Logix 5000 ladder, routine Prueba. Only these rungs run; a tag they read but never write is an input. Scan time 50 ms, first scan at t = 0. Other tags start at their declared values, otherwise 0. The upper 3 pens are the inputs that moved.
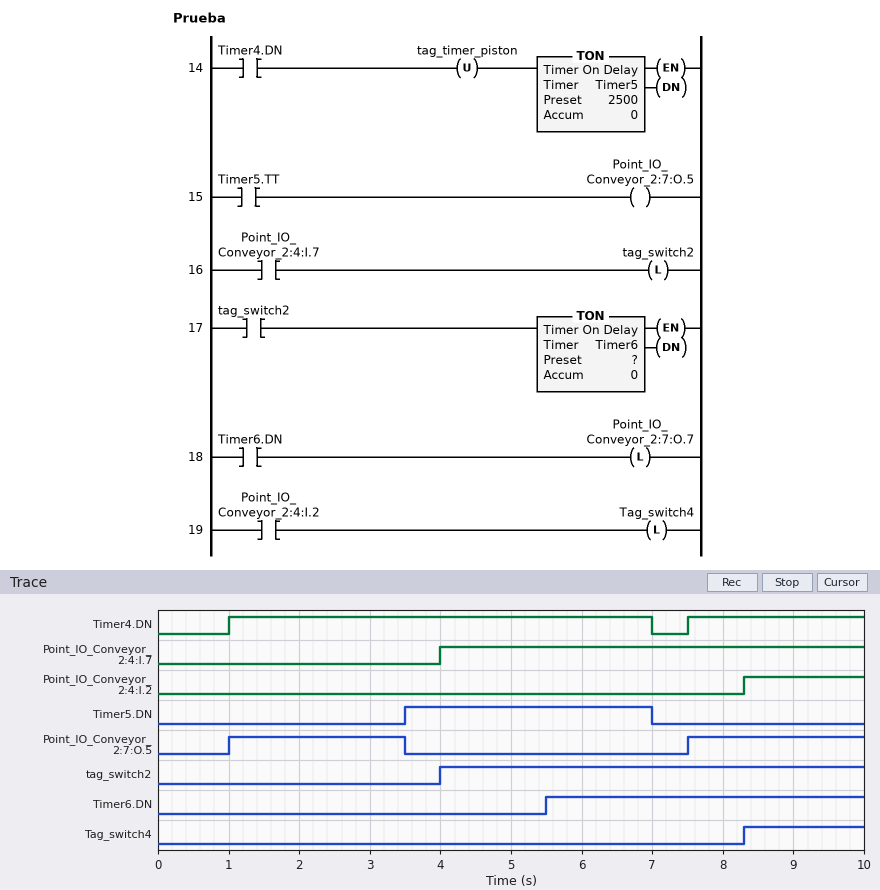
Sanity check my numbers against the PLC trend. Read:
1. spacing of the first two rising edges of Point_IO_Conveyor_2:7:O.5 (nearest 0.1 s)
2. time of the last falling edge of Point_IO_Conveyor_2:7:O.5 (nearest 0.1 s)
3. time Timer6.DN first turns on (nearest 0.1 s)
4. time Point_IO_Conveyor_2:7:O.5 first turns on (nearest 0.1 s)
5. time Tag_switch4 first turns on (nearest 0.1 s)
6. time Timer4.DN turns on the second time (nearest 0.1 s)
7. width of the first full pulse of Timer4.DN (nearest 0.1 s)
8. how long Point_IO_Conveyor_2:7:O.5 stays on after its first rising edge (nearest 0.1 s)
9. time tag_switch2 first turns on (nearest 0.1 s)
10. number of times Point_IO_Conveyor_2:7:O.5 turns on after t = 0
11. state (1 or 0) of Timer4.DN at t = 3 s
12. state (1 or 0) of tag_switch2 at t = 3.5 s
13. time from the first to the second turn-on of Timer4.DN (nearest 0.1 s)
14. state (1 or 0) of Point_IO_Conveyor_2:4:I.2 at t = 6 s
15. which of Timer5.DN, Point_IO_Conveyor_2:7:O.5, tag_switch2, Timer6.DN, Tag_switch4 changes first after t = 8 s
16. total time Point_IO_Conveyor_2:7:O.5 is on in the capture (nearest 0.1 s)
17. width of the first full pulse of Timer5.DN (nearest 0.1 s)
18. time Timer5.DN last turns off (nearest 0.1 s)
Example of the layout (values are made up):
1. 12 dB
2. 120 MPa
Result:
1. 6.5 s
2. 3.5 s
3. 5.5 s
4. 1.0 s
5. 8.3 s
6. 7.5 s
7. 6.0 s
8. 2.5 s
9. 4.0 s
10. 2
11. 1
12. 0
13. 6.5 s
14. 0
15. Tag_switch4
16. 5.0 s
17. 3.5 s
18. 7.0 s
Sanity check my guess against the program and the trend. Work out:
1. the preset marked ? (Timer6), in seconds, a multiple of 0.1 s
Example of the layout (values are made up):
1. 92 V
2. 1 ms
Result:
1. 1.5 s
